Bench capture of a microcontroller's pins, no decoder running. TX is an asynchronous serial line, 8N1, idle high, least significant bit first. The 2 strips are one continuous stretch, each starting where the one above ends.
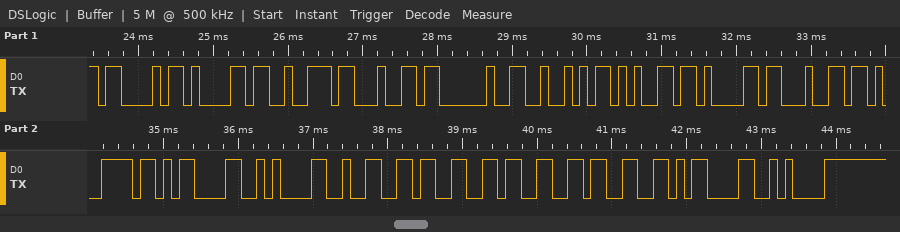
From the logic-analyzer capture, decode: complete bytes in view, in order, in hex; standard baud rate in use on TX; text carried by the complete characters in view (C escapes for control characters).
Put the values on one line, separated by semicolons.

43 61 72 64 20 52 65 61 64 79 0D 0A 32 33 33 33 0D 0A; 9600 baud; "Card Ready\r\n2333\r\n"
